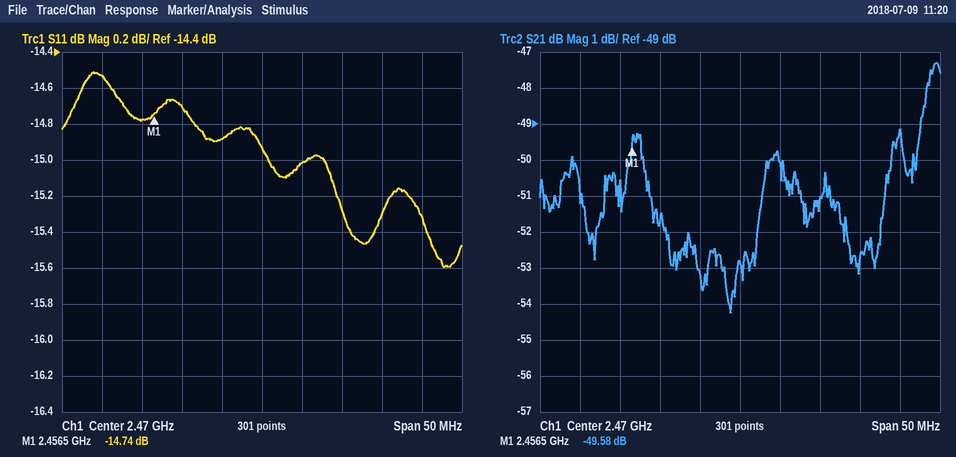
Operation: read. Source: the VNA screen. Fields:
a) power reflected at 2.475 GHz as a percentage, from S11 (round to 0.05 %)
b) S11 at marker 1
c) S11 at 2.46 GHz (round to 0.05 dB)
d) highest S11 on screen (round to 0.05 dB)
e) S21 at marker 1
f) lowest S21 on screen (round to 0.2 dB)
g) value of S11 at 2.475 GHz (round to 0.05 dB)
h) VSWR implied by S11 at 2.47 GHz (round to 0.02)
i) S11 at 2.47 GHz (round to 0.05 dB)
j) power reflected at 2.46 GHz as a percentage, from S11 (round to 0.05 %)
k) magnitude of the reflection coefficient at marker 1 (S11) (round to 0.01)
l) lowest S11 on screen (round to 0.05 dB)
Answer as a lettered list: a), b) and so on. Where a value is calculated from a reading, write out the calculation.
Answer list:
a) 10^(-15/10) ≈ 3.16 %, so 3.15 % to the nearest 0.05 %
b) -14.74 dB
c) -14.70 dB
d) -14.50 dB
e) -49.58 dB
f) -54.2 dB
g) -15.00 dB
h) |Γ| = 10^(-14.95/20) = 0.1789; VSWR = (1 + 0.1789)/(1 − 0.1789) ≈ 1.44
i) -14.95 dB
j) 10^(-14.7/10) ≈ 3.39 %, so 3.40 % to the nearest 0.05 %
k) 10^(-14.74/20) ≈ 0.18
l) -15.60 dB
